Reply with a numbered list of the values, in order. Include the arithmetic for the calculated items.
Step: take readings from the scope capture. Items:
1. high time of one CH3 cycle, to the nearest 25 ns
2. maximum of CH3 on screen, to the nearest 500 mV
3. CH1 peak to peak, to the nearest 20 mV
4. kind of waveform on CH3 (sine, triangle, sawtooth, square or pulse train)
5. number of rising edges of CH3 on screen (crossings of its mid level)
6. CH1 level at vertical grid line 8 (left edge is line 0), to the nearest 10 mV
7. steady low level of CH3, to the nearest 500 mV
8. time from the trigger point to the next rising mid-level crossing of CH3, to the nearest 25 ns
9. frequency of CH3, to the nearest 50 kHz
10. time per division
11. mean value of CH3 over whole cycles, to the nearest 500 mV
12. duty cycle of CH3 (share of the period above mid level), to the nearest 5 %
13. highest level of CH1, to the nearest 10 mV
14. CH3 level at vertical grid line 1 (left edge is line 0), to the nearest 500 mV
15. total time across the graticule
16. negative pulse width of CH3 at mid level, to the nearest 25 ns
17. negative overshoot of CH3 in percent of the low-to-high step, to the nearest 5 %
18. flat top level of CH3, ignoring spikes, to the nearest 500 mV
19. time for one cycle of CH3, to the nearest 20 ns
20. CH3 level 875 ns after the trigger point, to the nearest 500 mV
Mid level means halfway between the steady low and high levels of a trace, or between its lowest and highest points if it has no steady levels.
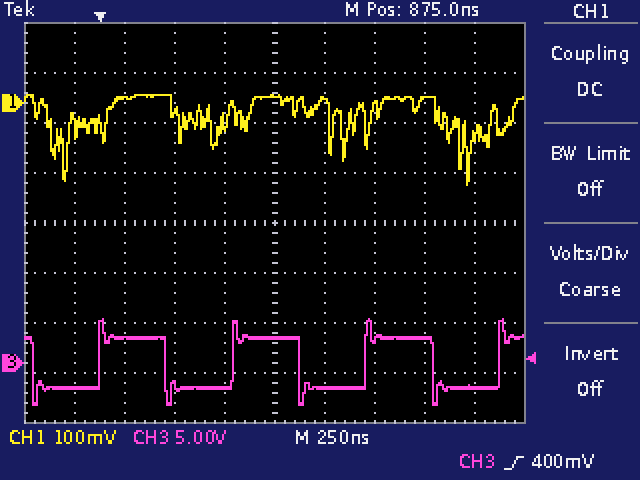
1. 325 ns
2. 4.5 V
3. 180 mV
4. square
5. 4
6. 10 mV
7. -2.5 V
8. 675 ns
9. 1 / 660 ns ≈ 1.52 MHz, so 1.50 MHz to the nearest 50 kHz
10. 250 ns
11. -2.5 V + 0.5 × (2.5 V − (-2.5 V)) ≈ 0.0 V
12. 325 ns / 660 ns ≈ 49.2 %, so 50 % to the nearest 5 %
13. 20 mV
14. -2.5 V
15. 2.5 µs
16. 325 ns
17. 35 %
18. 2.5 V
19. 660 ns
20. 2.5 V
